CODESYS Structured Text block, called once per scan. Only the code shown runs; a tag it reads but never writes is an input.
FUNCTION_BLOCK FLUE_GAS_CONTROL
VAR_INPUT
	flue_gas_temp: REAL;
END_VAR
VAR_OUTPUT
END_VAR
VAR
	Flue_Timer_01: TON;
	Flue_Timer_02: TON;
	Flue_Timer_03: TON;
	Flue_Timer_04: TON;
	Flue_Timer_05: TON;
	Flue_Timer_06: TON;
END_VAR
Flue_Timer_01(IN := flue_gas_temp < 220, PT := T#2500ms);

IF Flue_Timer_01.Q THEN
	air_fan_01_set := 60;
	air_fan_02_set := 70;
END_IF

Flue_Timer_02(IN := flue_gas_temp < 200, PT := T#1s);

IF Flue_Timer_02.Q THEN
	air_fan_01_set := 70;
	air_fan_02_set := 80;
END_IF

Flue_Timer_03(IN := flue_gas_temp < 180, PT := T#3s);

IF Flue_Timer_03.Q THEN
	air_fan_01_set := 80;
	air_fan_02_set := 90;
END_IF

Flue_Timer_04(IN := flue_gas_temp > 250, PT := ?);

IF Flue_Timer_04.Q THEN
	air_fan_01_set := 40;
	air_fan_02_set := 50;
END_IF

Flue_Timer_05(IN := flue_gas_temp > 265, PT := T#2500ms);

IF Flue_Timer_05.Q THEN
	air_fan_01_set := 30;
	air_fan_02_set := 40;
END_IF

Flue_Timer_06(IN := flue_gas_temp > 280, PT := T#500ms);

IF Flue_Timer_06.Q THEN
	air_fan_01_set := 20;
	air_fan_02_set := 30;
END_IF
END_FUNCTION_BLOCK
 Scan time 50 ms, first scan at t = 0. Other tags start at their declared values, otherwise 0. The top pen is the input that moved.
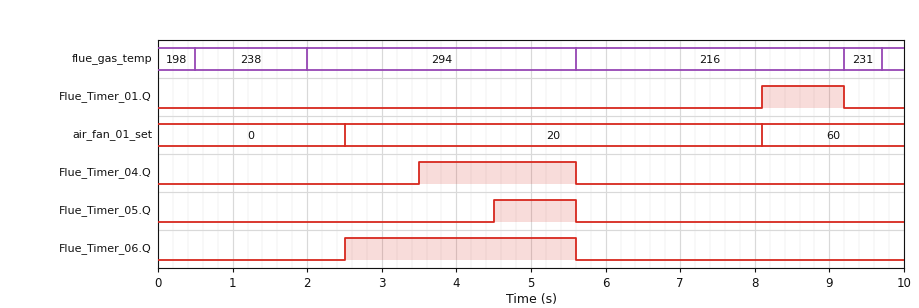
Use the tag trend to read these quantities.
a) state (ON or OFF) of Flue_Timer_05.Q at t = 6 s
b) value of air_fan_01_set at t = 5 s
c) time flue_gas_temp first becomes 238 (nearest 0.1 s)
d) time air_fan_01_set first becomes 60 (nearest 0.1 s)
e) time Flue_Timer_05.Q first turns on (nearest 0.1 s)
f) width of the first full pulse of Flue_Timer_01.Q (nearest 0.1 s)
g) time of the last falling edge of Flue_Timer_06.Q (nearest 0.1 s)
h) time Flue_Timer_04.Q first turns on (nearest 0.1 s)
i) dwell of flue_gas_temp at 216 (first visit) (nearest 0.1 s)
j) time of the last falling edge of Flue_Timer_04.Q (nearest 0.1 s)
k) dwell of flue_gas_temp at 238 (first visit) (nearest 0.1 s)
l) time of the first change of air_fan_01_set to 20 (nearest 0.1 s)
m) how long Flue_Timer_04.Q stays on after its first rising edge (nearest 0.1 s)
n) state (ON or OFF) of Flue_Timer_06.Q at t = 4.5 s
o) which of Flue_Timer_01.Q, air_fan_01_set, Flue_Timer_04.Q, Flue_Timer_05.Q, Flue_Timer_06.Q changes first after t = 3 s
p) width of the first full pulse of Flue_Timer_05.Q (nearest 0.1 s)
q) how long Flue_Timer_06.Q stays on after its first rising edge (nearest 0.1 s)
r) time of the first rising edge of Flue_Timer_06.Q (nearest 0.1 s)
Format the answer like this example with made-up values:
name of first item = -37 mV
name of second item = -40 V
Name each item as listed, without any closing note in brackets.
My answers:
state (ON or OFF) of Flue_Timer_05.Q at t = 6 s = OFF
value of air_fan_01_set at t = 5 s = 20
time flue_gas_temp first becomes 238 = 0.5 s
time air_fan_01_set first becomes 60 = 8.1 s
time Flue_Timer_05.Q first turns on = 4.5 s
width of the first full pulse of Flue_Timer_01.Q = 1.1 s
time of the last falling edge of Flue_Timer_06.Q = 5.6 s
time Flue_Timer_04.Q first turns on = 3.5 s
dwell of flue_gas_temp at 216 (first visit) = 3.6 s
time of the last falling edge of Flue_Timer_04.Q = 5.6 s
dwell of flue_gas_temp at 238 (first visit) = 1.5 s
time of the first change of air_fan_01_set to 20 = 2.5 s
how long Flue_Timer_04.Q stays on after its first rising edge = 2.1 s
state (ON or OFF) of Flue_Timer_06.Q at t = 4.5 s = ON
which of Flue_Timer_01.Q, air_fan_01_set, Flue_Timer_04.Q, Flue_Timer_05.Q, Flue_Timer_06.Q changes first after t = 3 s = Flue_Timer_04.Q
width of the first full pulse of Flue_Timer_05.Q = 1.1 s
how long Flue_Timer_06.Q stays on after its first rising edge = 3.1 s
time of the first rising edge of Flue_Timer_06.Q = 2.5 s
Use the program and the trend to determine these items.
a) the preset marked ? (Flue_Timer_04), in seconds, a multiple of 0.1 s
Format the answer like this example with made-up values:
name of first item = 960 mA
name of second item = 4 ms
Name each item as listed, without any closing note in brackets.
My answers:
the preset marked ? (Flue_Timer_04), in seconds, a multiple of 0.1 s = 1.5 s
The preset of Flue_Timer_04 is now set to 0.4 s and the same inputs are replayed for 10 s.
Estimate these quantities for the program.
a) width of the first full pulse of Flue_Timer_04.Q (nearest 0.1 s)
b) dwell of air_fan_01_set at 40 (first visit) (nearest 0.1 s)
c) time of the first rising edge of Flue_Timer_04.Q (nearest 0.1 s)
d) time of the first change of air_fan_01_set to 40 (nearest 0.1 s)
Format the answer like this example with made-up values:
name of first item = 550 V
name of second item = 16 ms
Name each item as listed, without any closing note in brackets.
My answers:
width of the first full pulse of Flue_Timer_04.Q = 3.2 s
dwell of air_fan_01_set at 40 (first visit) = 0.1 s
time of the first rising edge of Flue_Timer_04.Q = 2.4 s
time of the first change of air_fan_01_set to 40 = 2.4 s
